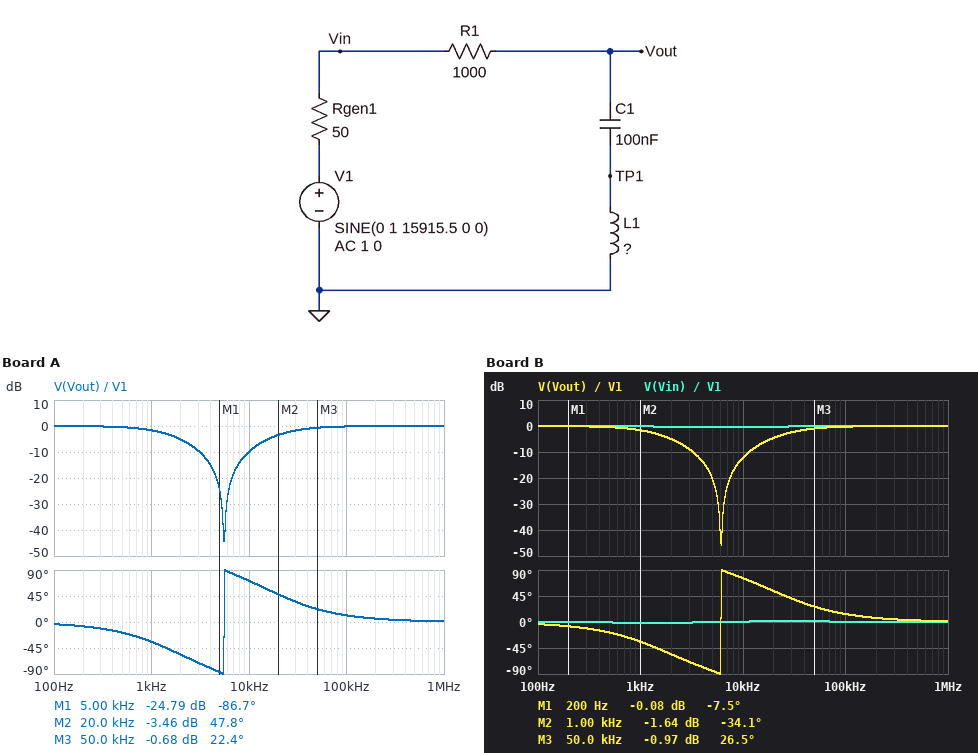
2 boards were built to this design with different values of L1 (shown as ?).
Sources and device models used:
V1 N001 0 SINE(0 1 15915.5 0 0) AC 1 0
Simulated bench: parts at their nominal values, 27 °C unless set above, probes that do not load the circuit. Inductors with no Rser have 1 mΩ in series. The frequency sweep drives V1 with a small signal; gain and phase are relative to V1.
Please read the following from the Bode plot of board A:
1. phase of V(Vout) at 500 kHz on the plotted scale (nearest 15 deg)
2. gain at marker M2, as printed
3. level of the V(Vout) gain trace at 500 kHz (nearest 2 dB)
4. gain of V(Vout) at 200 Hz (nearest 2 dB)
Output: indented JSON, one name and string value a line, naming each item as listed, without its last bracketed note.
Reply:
{
  "phase of V(Vout) at 500 kHz on the plotted scale": "0 deg",
  "gain at marker M2, as printed": "-3.46 dB",
  "level of the V(Vout) gain trace at 500 kHz": "0 dB",
  "gain of V(Vout) at 200 Hz": "0 dB"
}
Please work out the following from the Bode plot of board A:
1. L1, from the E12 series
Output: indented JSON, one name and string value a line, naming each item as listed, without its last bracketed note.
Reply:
{
  "L1, from the E12 series": "8.2 mH"
}
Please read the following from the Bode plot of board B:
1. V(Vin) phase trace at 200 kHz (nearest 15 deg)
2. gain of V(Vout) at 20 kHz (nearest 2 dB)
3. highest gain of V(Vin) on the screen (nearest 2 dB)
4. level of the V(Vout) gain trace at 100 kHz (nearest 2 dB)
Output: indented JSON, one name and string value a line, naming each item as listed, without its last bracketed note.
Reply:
{
  "V(Vin) phase trace at 200 kHz": "0 deg",
  "gain of V(Vout) at 20 kHz": "-4 dB",
  "highest gain of V(Vin) on the screen": "0 dB",
  "level of the V(Vout) gain trace at 100 kHz": "0 dB"
}
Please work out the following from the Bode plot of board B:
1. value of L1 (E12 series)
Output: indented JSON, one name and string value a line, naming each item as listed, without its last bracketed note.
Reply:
{
  "value of L1": "6.8 mH"
}
